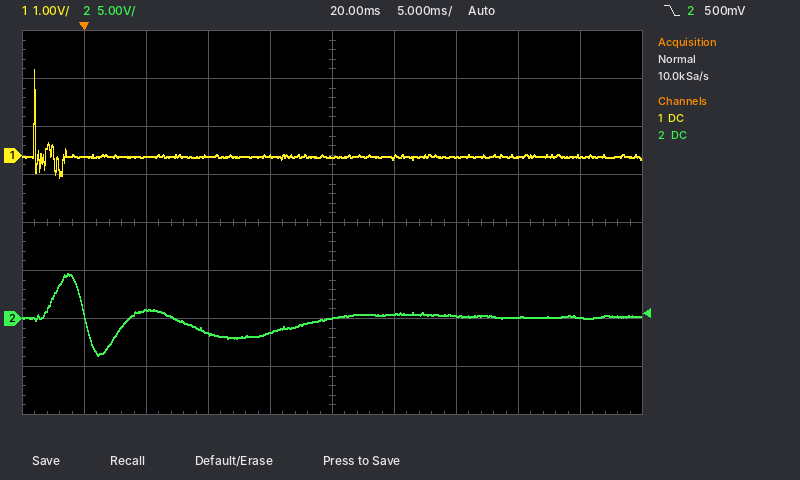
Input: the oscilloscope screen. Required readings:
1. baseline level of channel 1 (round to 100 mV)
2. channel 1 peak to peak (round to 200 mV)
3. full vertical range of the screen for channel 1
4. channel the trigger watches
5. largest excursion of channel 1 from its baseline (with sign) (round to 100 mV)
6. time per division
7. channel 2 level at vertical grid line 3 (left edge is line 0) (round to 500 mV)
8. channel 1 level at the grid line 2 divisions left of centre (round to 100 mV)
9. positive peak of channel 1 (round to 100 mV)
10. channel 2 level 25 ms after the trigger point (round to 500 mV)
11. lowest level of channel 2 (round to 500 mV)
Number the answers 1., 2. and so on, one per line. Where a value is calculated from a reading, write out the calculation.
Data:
1. 0.0 V
2. 2.2 V
3. 8 V
4. channel 2
5. 1.8 V − (0.0 V) = +1.8 V
6. 5 ms
7. -1.5 V
8. 0.0 V
9. 1.8 V
10. 500 mV
11. -4.0 V
